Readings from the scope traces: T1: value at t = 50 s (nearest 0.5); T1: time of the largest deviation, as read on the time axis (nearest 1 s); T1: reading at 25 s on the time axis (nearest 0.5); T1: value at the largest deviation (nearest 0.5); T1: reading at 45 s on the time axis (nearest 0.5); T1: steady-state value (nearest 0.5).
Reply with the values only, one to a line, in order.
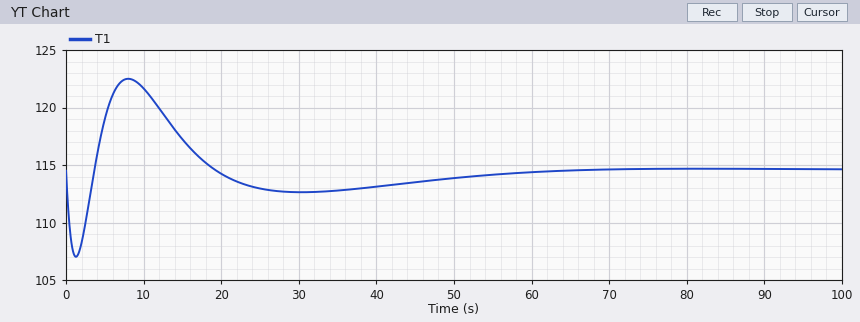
114.0
8 s
113.0
122.5
113.5
114.5
